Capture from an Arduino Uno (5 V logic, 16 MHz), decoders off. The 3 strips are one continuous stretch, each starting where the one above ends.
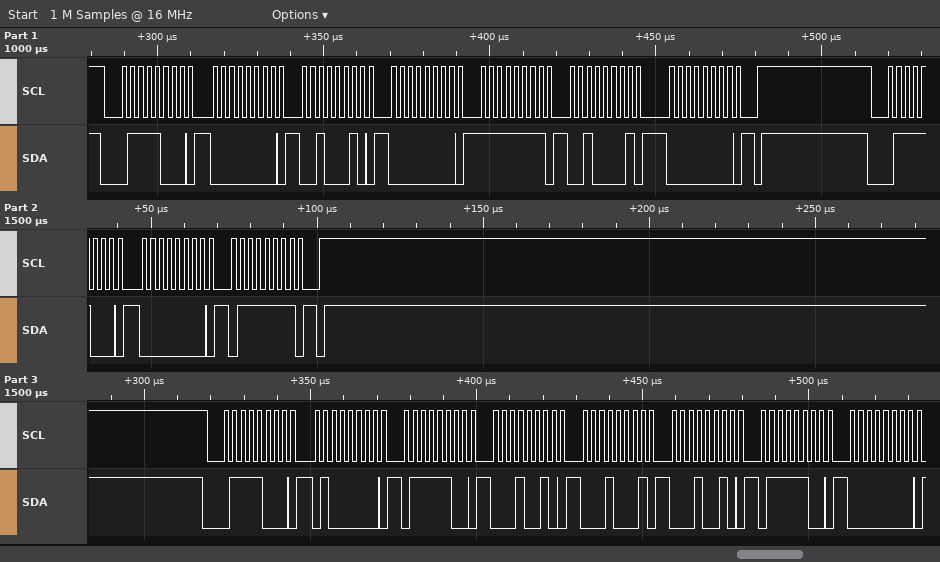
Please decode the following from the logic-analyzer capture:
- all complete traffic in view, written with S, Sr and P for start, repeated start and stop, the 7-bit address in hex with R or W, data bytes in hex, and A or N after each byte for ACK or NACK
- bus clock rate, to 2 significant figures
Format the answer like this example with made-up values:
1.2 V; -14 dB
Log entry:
S 3CW A 00 A 22 A 00 A FF A 21 A 00 A P S 3CW A 00 A 7F A P S 3CW A 40 A 7C A 12 A 11 A 12 A 7C A 00 A; 400 kHz
